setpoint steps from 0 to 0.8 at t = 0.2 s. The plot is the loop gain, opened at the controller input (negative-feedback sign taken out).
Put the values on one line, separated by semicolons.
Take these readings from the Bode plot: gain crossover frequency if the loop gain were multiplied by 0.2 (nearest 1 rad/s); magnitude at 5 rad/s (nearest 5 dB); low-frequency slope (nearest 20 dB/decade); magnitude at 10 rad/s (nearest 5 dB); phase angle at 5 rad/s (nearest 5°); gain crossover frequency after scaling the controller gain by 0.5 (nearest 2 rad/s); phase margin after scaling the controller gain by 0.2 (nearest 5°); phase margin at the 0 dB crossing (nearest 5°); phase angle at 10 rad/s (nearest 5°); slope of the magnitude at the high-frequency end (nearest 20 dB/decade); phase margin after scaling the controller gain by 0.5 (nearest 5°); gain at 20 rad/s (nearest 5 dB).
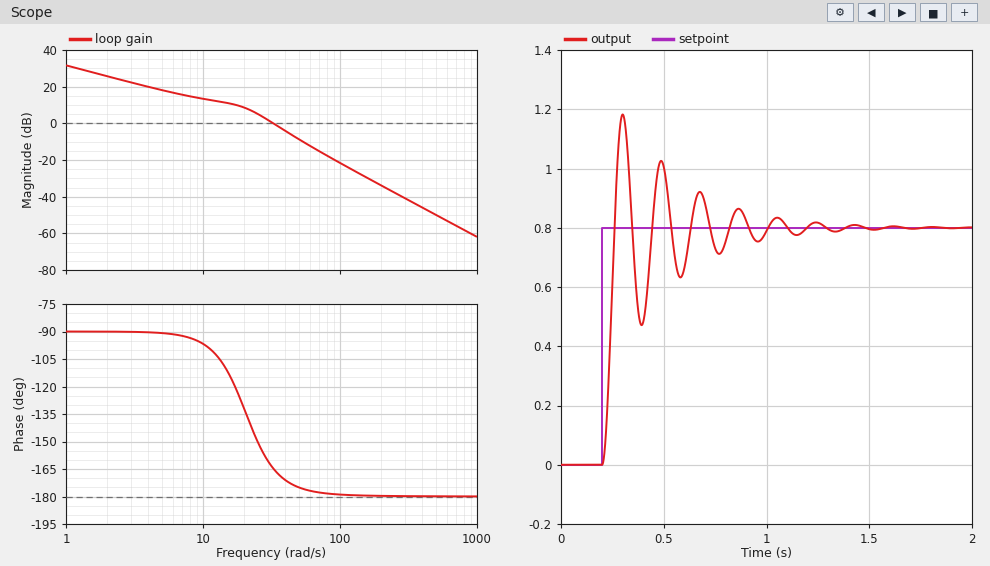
9 rad/s; 20 dB; -20 dB/decade; 15 dB; -90°; 24 rad/s; 85°; 15°; -95°; -40 dB/decade; 35°; 10 dB
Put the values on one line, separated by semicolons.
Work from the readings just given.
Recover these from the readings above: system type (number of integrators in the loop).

1
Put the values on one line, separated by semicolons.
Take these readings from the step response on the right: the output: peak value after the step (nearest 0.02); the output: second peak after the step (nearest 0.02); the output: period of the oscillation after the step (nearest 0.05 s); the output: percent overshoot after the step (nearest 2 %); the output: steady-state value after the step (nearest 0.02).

1.18; 1.02; 0.20 s; 48 %; 0.80
